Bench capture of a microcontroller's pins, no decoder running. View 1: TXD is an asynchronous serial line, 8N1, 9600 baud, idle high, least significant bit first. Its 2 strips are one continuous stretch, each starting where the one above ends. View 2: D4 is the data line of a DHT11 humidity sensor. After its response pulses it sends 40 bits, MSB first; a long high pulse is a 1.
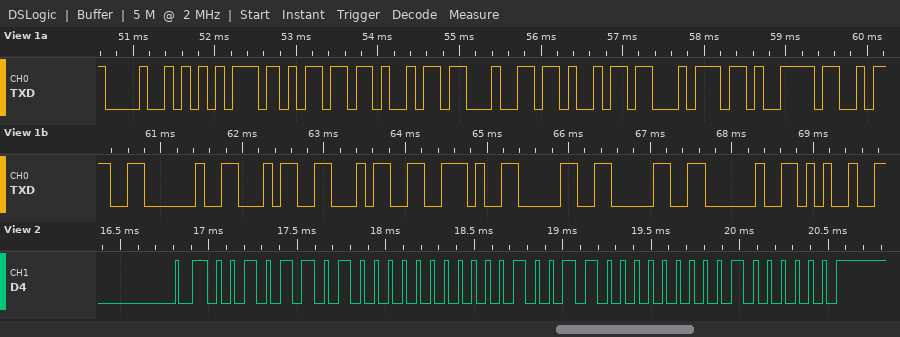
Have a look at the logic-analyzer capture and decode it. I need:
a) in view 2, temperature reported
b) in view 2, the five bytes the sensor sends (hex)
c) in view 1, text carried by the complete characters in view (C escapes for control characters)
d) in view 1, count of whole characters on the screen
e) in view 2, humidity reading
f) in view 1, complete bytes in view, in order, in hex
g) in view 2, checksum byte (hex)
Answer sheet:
19.0 °C
2D 00 13 00 40
"Humidity: 44.00 %"
17
45 %
48 75 6D 69 64 69 74 79 3A 20 34 34 2E 30 30 20 25
0x40
